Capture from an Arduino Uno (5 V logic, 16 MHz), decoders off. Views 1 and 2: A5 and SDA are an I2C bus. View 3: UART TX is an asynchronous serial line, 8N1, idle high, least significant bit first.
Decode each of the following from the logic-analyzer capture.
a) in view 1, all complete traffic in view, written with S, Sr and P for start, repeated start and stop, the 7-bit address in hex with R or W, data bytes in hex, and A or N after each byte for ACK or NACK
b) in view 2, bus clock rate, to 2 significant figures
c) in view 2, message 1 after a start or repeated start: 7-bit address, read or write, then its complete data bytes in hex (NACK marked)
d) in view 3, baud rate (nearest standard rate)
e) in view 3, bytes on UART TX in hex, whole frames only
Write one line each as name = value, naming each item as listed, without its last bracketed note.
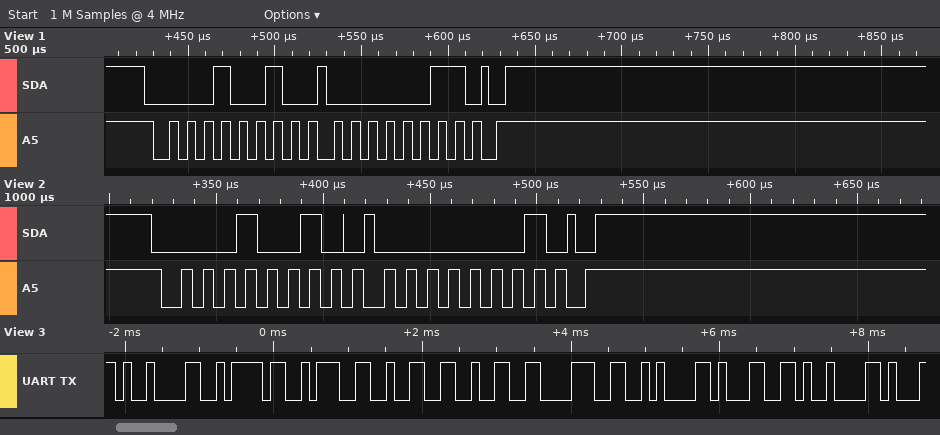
in view 1, all complete traffic in view, written with S, Sr and P for start, repeated start and stop, the 7-bit address in hex with R or W, data bytes in hex, and A or N after each byte for ACK or NACK = S 09W A 03 A P
in view 2, bus clock rate, to 2 significant figures = 100 kHz
in view 2, message 1 after a start or repeated start: 7-bit address, read or write, then its complete data bytes in hex = 0x09 write: 01
in view 3, baud rate = 9600 baud
in view 3, bytes on UART TX in hex, whole frames only = 0x09 0x7A 0x3A 0x32 0x32 0x38 0x0A 0x31 0x09
